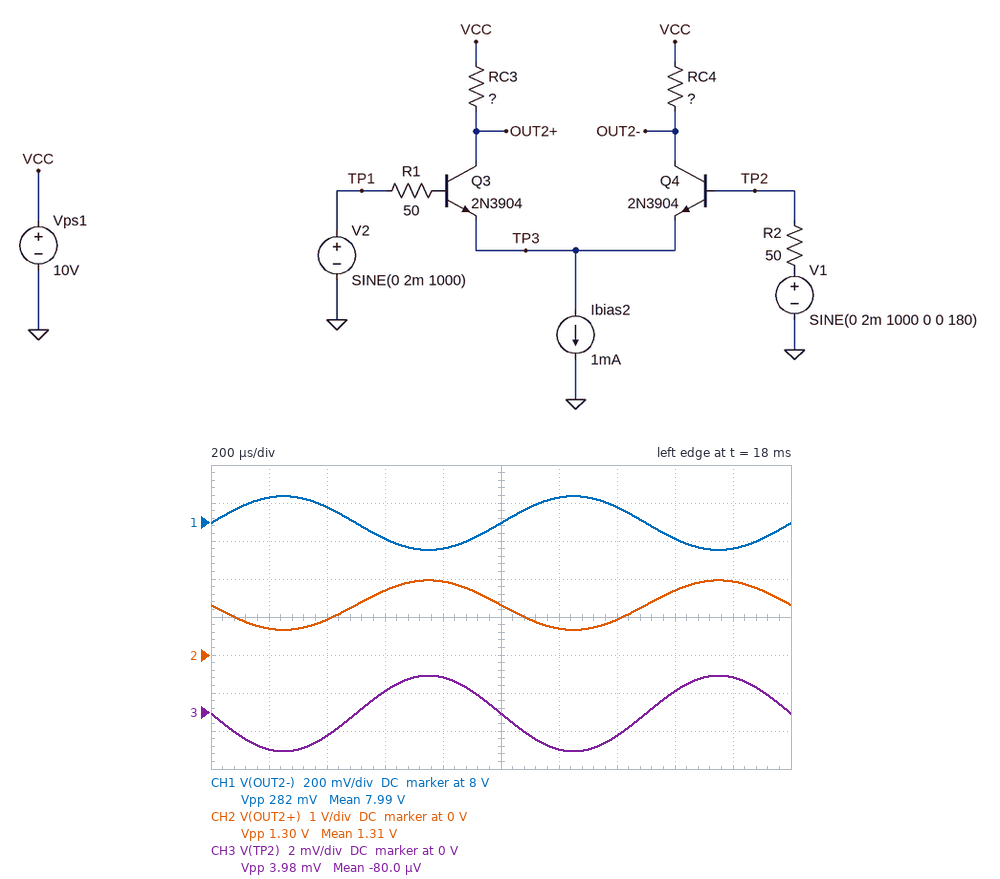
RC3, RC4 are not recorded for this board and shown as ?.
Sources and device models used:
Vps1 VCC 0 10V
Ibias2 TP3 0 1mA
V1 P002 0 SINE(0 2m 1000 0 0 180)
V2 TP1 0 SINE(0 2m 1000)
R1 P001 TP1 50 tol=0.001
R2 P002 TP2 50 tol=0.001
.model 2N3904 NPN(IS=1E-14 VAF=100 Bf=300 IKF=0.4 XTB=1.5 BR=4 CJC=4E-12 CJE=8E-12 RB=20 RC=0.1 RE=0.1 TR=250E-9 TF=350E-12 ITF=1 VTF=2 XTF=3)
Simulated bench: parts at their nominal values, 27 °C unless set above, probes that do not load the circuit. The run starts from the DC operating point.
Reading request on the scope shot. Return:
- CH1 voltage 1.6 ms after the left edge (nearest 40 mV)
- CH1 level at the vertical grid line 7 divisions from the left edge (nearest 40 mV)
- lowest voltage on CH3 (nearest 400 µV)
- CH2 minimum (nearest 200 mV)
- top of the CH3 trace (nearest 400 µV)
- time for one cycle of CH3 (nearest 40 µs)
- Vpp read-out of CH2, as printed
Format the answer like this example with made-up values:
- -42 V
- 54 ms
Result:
- 7.92 V
- 8.08 V
- -2.0 mV
- 600 mV
- 2.0 mV
- 1.00 ms
- 1.30 V
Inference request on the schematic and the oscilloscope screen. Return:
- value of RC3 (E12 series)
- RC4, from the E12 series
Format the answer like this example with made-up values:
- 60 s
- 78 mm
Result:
- 18 kΩ
- 3.9 kΩ
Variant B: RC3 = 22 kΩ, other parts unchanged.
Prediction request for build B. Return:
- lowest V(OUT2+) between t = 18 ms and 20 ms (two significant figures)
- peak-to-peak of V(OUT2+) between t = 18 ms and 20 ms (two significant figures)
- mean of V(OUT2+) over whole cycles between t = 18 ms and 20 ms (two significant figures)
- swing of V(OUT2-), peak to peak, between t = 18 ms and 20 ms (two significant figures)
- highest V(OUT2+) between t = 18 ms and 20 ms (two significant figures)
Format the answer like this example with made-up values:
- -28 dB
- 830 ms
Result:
- -570 mV
- 840 mV
- -280 mV
- 190 mV
- 270 mV
